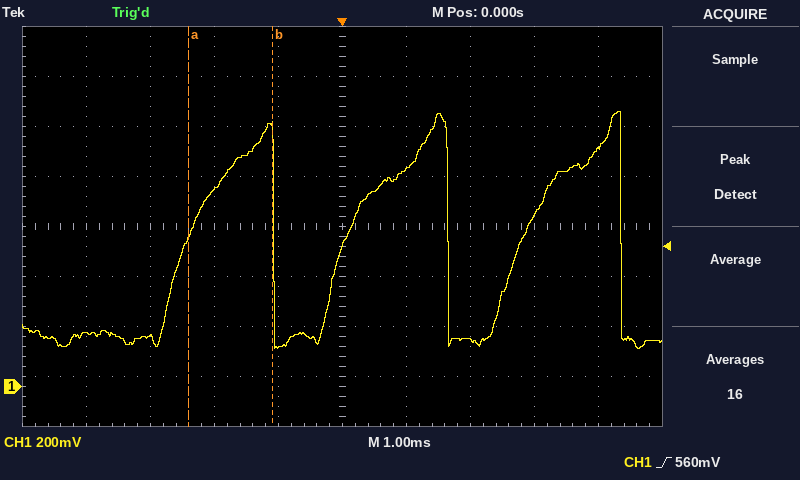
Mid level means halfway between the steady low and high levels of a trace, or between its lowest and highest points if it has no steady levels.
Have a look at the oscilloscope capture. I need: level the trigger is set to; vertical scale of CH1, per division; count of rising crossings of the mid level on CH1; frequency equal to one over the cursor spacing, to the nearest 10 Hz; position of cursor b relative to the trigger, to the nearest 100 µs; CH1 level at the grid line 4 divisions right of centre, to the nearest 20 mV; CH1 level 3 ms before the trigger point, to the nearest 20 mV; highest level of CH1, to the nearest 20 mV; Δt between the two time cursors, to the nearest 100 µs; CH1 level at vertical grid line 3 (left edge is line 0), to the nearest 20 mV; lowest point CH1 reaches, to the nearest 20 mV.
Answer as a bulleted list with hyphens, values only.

- 560 mV
- 200 mV
- 3
- 770 Hz
- -1.1 ms
- 960 mV
- 200 mV
- 1.10 V
- 1.3 ms
- 780 mV
- 160 mV
